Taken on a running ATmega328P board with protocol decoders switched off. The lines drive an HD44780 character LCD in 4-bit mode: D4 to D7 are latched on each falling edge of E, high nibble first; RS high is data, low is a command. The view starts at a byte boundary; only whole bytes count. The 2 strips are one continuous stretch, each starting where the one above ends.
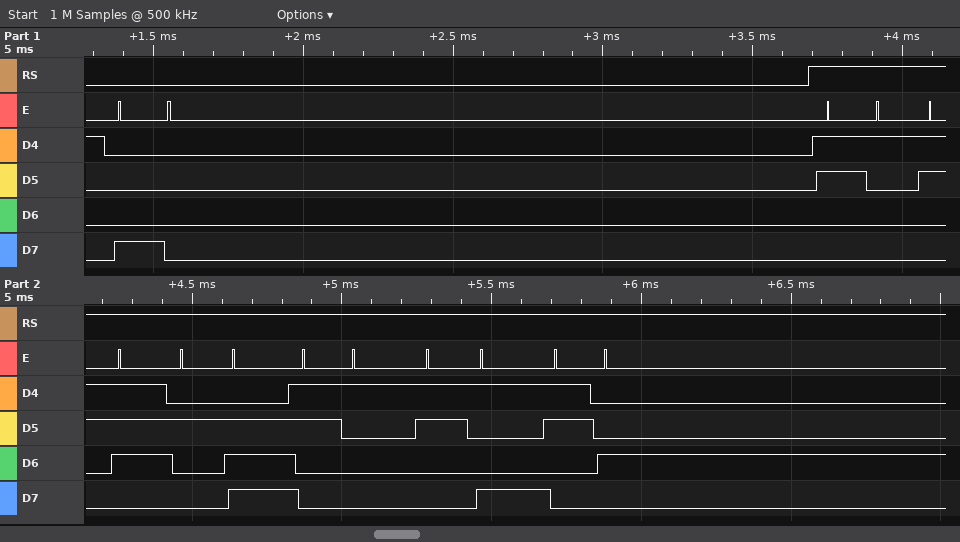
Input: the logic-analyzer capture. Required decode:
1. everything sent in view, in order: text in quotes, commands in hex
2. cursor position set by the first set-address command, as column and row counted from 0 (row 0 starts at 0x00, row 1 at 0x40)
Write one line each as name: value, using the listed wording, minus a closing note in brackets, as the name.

everything sent in view, in order: text in quotes, commands in hex: 0x80 "17.194"
cursor position set by the first set-address command, as column and row counted from 0: column 0, row 0
